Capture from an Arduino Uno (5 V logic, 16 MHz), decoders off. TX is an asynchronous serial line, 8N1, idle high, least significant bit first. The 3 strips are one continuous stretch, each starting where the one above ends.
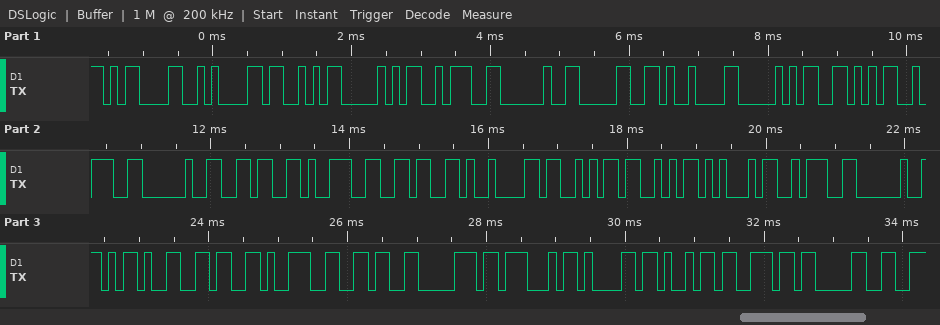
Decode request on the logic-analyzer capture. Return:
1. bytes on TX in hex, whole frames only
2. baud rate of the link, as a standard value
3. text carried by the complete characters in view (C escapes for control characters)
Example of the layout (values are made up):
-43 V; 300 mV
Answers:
0D 0A 53 50 3A 20 30 09 50 56 3A 20 36 39 36 09 53 53 45 3A 20 2D 36 39 36 70 47 61 69 6E 30; 9600 baud; "\r\nSP: 0\tPV: 696\tSSE: -696pGain0"
